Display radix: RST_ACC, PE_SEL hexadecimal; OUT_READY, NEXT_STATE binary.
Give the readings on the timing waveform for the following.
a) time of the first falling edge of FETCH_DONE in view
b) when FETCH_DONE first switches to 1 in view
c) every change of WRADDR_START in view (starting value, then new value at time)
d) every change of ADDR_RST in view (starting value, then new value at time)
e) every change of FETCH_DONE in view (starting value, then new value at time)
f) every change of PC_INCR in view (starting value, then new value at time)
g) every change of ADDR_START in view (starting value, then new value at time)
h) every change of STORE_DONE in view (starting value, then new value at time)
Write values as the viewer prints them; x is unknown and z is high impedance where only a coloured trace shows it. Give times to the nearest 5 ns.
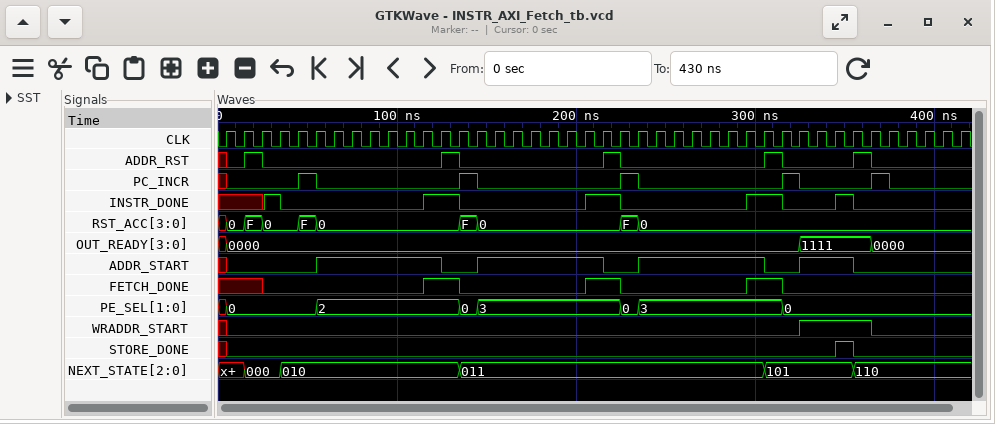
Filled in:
135 ns
115 ns
x, 0 at 5 ns, 1 at 325 ns, 0 at 365 ns
x, 0 at 5 ns, 1 at 15 ns, 0 at 25 ns, 1 at 125 ns, 0 at 135 ns, 1 at 215 ns, 0 at 225 ns, 1 at 305 ns, 0 at 315 ns, 1 at 355 ns, 0 at 365 ns
x, 0 at 25 ns, 1 at 115 ns, 0 at 135 ns, 1 at 205 ns, 0 at 225 ns, 1 at 295 ns, 0 at 315 ns
x, 0 at 5 ns, 1 at 45 ns, 0 at 55 ns, 1 at 135 ns, 0 at 145 ns, 1 at 225 ns, 0 at 235 ns, 1 at 315 ns, 0 at 325 ns, 1 at 365 ns, 0 at 375 ns
x, 0 at 5 ns, 1 at 55 ns, 0 at 125 ns, 1 at 145 ns, 0 at 215 ns, 1 at 235 ns, 0 at 305 ns, 1 at 325 ns, 0 at 355 ns
x, 0 at 5 ns, 1 at 345 ns, 0 at 355 ns
